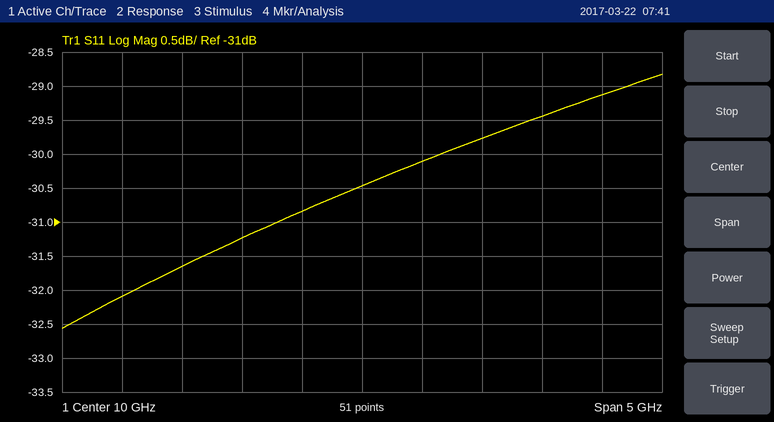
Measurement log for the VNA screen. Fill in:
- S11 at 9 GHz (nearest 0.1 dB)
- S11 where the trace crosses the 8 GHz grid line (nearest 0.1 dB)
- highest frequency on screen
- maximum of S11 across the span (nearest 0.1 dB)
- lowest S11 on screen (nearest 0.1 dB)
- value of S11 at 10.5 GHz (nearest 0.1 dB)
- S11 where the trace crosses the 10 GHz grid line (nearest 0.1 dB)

-31.2 dB
-32.1 dB
12.5 GHz
-28.8 dB
-32.6 dB
-30.1 dB
-30.5 dB
